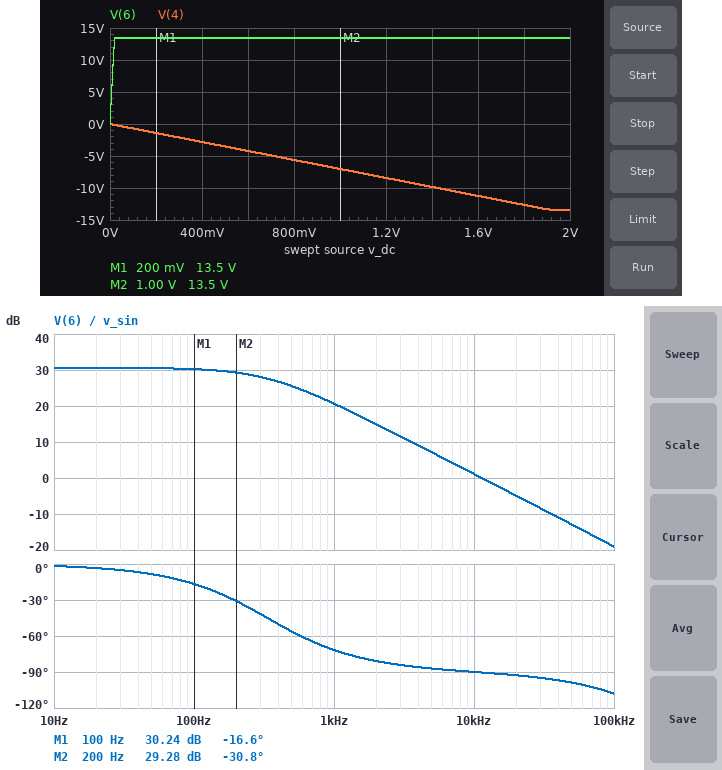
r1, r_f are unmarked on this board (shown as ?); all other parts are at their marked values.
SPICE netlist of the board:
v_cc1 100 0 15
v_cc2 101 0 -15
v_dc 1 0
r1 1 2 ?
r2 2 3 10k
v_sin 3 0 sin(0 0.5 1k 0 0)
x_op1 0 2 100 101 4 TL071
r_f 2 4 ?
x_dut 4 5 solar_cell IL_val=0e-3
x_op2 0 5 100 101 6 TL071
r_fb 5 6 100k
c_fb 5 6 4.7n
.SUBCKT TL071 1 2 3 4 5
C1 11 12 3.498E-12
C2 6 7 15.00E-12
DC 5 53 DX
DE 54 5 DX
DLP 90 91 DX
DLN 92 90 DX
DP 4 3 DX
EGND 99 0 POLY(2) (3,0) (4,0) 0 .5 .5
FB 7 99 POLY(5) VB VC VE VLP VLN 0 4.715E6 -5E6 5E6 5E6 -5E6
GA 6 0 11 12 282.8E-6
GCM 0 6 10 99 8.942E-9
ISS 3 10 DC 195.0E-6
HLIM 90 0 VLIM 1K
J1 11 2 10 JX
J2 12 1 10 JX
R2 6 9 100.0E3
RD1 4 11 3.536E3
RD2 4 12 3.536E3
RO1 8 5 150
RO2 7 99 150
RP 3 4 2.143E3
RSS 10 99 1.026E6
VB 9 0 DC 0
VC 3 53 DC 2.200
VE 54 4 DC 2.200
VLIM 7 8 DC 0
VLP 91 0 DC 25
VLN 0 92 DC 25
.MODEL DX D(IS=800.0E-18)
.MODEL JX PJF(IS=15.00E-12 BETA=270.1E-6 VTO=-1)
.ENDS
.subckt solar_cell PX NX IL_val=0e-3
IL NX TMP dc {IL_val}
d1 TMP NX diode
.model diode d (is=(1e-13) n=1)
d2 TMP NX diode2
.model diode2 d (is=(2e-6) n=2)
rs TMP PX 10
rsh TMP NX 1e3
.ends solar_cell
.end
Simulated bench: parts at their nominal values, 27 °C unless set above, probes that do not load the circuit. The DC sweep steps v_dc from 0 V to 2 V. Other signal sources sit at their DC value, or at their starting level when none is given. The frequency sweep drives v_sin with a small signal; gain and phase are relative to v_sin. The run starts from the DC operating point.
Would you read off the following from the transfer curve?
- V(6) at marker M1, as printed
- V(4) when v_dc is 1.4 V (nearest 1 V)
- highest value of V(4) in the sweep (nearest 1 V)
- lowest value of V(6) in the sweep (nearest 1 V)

13.5 V
-10 V
0 V
0 V
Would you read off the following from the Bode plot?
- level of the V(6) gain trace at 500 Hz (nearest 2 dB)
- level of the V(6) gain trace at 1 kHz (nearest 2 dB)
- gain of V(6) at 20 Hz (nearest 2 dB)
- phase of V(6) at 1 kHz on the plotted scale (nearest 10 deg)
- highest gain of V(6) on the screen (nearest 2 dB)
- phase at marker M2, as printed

26 dB
20 dB
30 dB
-70 deg
30 dB
-30.8 deg
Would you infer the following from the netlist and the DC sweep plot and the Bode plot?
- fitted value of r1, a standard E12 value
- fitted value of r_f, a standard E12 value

470 Ω
3.3 kΩ
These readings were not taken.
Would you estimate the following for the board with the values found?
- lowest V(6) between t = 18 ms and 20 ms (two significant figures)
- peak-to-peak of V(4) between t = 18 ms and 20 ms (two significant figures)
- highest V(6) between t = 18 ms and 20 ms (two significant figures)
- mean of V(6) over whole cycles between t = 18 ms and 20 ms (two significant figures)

-6.7 V
330 mV
4.8 V
-880 mV
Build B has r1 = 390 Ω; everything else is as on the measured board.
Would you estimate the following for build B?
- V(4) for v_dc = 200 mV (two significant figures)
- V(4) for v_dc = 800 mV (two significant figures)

-1.7 V
-6.8 V
